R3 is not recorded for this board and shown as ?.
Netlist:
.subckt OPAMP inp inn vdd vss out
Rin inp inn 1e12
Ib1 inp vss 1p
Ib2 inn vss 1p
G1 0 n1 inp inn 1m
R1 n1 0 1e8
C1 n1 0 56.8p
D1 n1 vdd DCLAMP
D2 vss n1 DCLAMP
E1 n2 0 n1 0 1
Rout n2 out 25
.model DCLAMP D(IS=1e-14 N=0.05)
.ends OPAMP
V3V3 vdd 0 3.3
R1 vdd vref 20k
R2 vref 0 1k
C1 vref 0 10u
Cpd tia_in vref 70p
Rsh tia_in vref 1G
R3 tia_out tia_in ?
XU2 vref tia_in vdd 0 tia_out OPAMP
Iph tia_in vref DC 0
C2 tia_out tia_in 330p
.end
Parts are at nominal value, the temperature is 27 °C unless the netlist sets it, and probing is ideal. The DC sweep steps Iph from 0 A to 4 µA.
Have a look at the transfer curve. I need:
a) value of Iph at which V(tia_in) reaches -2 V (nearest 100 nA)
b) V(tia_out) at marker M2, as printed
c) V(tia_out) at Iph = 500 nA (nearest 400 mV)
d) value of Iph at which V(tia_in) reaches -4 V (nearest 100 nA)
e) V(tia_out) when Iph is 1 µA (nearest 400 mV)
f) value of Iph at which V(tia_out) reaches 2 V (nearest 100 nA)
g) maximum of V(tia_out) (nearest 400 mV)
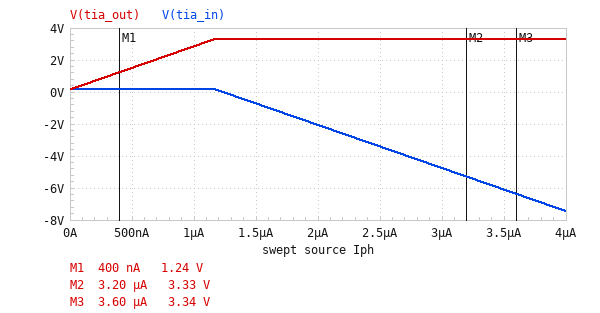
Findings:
2.0 µA
3.33 V
1.6 V
2.7 µA
2.8 V
700 nA
3.2 V
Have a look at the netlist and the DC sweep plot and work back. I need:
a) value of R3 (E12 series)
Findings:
2.7 MΩ
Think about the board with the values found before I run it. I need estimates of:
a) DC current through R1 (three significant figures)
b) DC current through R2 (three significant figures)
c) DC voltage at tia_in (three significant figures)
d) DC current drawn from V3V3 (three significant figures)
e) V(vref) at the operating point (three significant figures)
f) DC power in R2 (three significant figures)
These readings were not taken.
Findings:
157 µA
157 µA
157 mV
157 µA
157 mV
24.7 µW
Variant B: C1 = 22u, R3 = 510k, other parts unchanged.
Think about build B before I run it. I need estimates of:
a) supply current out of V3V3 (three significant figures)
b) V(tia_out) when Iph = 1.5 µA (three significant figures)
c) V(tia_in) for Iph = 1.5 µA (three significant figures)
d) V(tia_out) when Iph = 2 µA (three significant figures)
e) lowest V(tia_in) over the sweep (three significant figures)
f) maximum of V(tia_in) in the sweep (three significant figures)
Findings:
157 µA
924 mV
159 mV
1.18 V
157 mV
161 mV
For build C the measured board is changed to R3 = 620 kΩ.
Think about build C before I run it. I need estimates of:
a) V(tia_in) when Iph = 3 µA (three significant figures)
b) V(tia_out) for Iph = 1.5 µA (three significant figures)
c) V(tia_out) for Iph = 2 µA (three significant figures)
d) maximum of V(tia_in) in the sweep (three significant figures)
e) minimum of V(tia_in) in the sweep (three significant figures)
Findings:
160 mV
1.09 V
1.40 V
161 mV
157 mV
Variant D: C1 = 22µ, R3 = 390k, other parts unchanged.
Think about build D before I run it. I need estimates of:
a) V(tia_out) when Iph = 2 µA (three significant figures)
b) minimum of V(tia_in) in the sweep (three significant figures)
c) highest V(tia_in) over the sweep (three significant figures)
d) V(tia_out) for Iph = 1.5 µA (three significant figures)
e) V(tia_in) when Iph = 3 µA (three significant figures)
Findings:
939 mV
157 mV
161 mV
744 mV
160 mV
